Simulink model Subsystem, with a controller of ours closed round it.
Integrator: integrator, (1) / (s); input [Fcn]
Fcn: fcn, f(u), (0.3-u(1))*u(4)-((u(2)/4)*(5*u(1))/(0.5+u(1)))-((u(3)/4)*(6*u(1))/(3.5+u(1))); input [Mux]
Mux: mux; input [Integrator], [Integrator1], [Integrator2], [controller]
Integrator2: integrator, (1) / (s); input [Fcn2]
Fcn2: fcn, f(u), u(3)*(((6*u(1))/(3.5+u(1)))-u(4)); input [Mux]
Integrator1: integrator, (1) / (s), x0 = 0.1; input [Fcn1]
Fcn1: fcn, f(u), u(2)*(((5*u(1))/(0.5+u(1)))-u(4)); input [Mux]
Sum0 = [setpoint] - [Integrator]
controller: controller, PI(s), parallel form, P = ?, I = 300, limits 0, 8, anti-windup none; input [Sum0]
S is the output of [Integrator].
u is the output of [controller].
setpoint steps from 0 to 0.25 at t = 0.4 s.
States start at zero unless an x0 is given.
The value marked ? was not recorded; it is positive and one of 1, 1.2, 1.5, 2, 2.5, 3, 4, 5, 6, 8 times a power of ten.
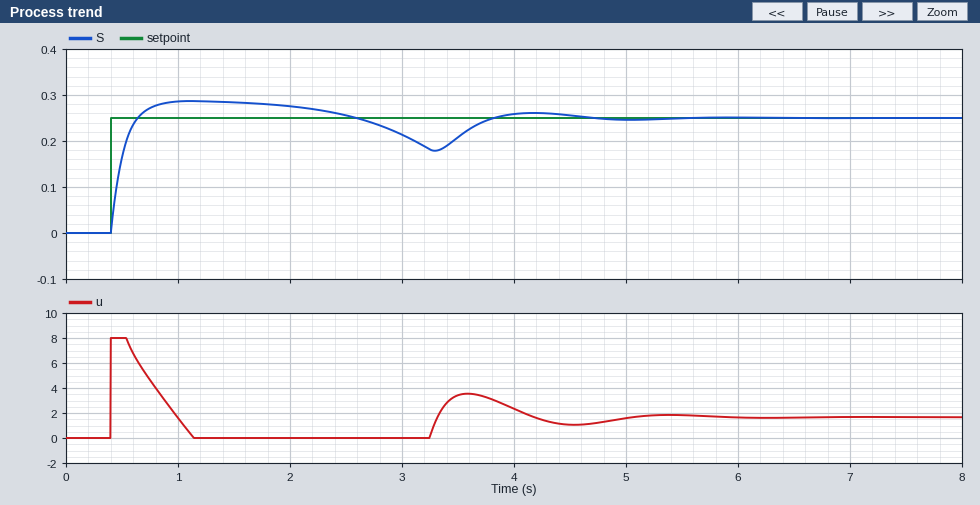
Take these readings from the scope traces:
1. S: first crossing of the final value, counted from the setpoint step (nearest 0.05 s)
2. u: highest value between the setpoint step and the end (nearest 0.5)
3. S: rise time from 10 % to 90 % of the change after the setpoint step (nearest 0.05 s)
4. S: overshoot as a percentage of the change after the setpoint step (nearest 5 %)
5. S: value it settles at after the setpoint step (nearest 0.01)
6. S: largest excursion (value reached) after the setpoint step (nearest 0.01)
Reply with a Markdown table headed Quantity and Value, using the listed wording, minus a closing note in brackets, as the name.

| Quantity | Value |
|---|---|
| S: first crossing of the final value, counted from the setpoint step | 0.25 s |
| u: highest value between the setpoint step and the end | 8.0 |
| S: rise time from 10 % to 90 % of the change after the setpoint step | 0.15 s |
| S: overshoot as a percentage of the change after the setpoint step | 15 % |
| S: value it settles at after the setpoint step | 0.25 |
| S: largest excursion (value reached) after the setpoint step | 0.29 |
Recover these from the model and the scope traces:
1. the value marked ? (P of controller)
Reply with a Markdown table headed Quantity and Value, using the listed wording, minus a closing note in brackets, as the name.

| Quantity | Value |
|---|---|
| the value marked ? | 50 |
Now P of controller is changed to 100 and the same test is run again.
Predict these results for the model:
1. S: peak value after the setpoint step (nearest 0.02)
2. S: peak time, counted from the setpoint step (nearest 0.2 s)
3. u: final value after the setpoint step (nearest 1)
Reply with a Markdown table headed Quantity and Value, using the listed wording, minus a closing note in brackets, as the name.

| Quantity | Value |
|---|---|
| S: peak value after the setpoint step | 0.28 |
| S: peak time, counted from the setpoint step | 0.6 s |
| u: final value after the setpoint step | 2 |
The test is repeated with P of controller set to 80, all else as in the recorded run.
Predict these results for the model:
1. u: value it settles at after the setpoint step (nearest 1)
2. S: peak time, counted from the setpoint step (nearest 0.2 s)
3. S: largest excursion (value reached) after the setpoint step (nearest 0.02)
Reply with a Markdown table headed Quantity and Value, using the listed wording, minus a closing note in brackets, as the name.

| Quantity | Value |
|---|---|
| u: value it settles at after the setpoint step | 2 |
| S: peak time, counted from the setpoint step | 0.6 s |
| S: largest excursion (value reached) after the setpoint step | 0.28 |
